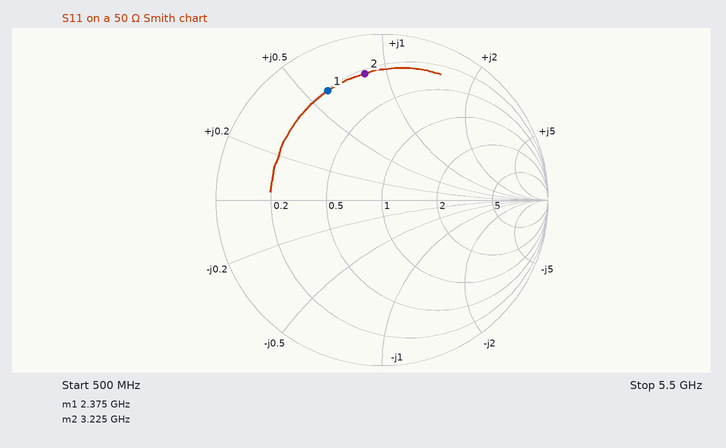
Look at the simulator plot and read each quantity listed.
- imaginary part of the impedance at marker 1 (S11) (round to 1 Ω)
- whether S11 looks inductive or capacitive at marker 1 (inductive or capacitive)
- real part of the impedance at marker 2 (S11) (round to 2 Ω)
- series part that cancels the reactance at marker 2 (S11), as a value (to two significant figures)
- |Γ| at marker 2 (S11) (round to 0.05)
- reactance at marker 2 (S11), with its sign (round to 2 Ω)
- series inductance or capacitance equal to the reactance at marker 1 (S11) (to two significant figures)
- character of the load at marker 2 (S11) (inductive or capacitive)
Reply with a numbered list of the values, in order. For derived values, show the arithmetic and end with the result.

1. +30 Ω
2. inductive
3. 12 Ω
4. C = 1/(2π × 3.225 GHz × 42 Ω) ≈ 1.2 pF
5. 0.75
6. +42 Ω
7. L = 30 Ω/(2π × 2.375 GHz) ≈ 2.0 nH
8. inductive
